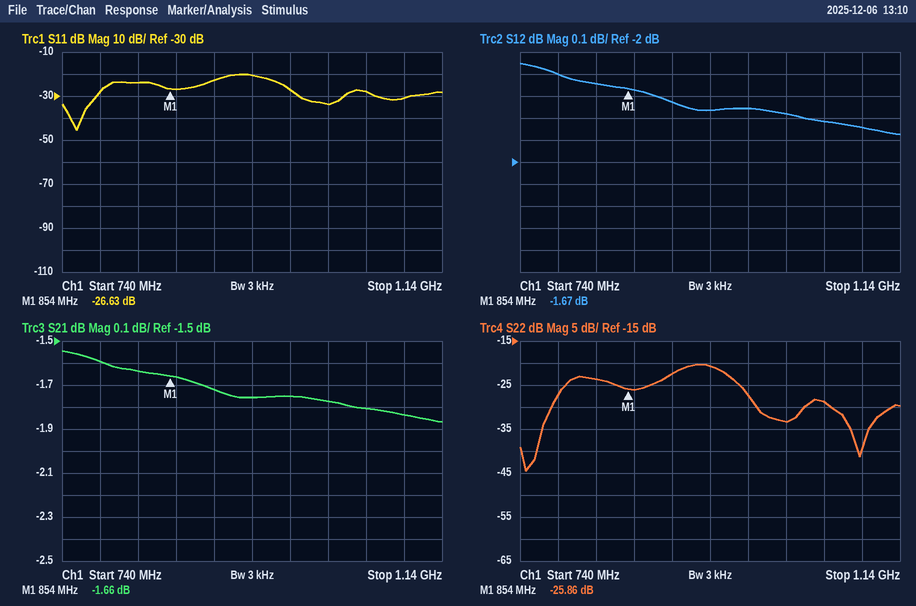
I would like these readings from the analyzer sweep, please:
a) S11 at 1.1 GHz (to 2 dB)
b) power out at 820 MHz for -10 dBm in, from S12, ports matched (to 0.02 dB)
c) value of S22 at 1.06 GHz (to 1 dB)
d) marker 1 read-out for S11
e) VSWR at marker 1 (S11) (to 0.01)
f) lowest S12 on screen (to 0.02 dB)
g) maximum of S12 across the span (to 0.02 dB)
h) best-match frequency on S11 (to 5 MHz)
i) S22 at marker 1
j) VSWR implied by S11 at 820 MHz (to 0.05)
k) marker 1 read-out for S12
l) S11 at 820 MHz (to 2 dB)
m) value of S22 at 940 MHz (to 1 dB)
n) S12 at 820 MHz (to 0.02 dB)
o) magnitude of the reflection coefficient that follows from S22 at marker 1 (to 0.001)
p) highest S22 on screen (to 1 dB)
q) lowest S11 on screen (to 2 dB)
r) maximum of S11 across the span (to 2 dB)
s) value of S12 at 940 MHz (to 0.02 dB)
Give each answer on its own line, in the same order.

-30 dB
-11.64 dBm
-29 dB
-26.63 dB
1.10
-1.88 dB
-1.56 dB
755 MHz
-25.86 dB
1.15
-1.67 dB
-24 dB
-21 dB
-1.64 dB
0.051
-20 dB
-46 dB
-20 dB
-1.76 dB
